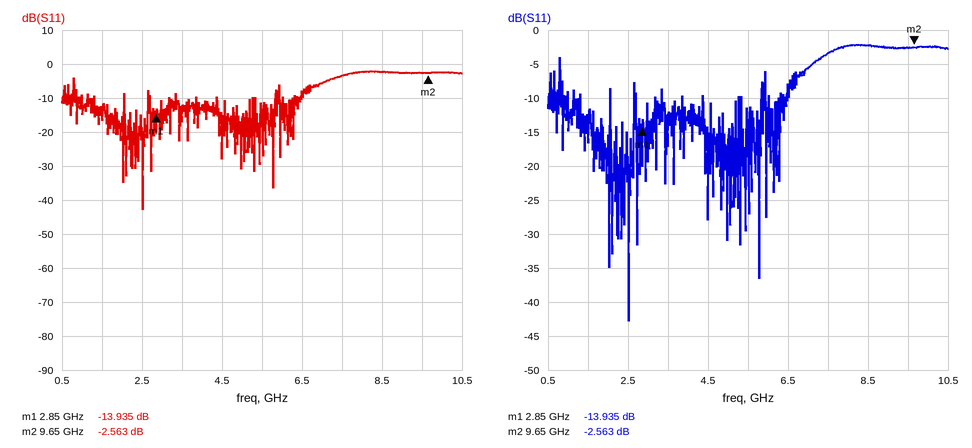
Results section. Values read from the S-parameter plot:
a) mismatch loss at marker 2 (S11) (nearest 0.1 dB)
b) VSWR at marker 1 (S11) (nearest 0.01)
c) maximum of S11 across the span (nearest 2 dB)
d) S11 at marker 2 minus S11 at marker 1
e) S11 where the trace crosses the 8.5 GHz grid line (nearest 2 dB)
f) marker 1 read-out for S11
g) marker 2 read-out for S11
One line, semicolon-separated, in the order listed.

3.5 dB; 1.50; -2 dB; 11.372 dB; -2 dB; -13.935 dB; -2.563 dB
